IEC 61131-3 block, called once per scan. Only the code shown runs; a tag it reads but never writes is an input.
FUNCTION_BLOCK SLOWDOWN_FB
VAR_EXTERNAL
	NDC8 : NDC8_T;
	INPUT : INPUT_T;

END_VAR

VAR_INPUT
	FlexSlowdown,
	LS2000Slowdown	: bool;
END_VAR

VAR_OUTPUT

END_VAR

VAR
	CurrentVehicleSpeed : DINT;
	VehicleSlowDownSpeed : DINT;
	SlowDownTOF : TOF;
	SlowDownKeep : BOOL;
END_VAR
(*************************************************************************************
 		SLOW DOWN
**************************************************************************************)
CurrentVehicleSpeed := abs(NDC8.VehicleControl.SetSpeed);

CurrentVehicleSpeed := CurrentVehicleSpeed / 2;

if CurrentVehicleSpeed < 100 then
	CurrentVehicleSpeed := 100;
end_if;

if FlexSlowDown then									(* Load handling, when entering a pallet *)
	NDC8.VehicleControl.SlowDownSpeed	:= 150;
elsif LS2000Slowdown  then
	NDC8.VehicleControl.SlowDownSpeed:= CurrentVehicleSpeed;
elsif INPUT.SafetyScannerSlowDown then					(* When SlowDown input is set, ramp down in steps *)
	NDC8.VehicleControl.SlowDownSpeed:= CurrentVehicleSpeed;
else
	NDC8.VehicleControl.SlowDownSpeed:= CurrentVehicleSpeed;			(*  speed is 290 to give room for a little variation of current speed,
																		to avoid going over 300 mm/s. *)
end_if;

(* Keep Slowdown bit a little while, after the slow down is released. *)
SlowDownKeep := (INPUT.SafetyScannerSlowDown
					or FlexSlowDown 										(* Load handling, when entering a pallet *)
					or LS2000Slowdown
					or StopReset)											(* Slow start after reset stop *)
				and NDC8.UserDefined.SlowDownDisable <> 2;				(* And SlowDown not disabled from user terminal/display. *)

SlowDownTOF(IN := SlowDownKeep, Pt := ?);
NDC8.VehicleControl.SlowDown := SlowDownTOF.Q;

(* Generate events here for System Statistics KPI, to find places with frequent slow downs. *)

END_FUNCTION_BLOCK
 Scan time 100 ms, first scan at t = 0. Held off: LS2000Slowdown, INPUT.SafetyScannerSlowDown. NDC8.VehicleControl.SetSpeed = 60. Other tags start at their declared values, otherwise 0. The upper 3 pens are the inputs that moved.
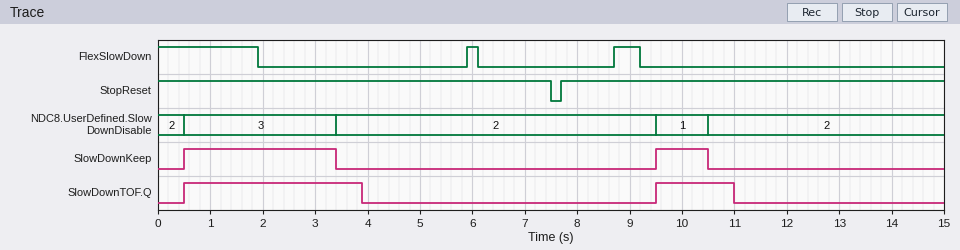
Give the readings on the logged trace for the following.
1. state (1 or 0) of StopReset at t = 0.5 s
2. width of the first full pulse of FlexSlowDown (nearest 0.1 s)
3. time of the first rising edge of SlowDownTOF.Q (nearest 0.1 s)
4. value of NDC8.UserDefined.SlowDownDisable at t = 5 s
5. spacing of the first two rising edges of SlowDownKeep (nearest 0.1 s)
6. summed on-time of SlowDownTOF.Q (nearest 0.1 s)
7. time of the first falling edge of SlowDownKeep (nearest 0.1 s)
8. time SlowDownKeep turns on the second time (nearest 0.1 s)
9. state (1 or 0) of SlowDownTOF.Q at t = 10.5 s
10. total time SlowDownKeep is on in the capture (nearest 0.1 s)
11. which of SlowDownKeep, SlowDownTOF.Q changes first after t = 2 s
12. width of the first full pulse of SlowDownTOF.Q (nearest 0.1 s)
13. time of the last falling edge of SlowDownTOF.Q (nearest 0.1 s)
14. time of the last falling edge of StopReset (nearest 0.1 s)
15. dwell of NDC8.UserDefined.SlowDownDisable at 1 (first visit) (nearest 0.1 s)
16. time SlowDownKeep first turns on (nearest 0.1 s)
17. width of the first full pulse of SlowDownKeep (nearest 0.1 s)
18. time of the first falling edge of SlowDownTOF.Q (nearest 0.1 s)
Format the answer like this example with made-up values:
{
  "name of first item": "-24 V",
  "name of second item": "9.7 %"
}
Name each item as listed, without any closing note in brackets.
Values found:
{
  "state (1 or 0) of StopReset at t = 0.5 s": "1",
  "width of the first full pulse of FlexSlowDown": "0.2 s",
  "time of the first rising edge of SlowDownTOF.Q": "0.5 s",
  "value of NDC8.UserDefined.SlowDownDisable at t = 5 s": "2",
  "spacing of the first two rising edges of SlowDownKeep": "9.0 s",
  "summed on-time of SlowDownTOF.Q": "4.9 s",
  "time of the first falling edge of SlowDownKeep": "3.4 s",
  "time SlowDownKeep turns on the second time": "9.5 s",
  "state (1 or 0) of SlowDownTOF.Q at t = 10.5 s": "1",
  "total time SlowDownKeep is on in the capture": "3.9 s",
  "which of SlowDownKeep, SlowDownTOF.Q changes first after t = 2 s": "SlowDownKeep",
  "width of the first full pulse of SlowDownTOF.Q": "3.4 s",
  "time of the last falling edge of SlowDownTOF.Q": "11.0 s",
  "time of the last falling edge of StopReset": "7.5 s",
  "dwell of NDC8.UserDefined.SlowDownDisable at 1 (first visit)": "1.0 s",
  "time SlowDownKeep first turns on": "0.5 s",
  "width of the first full pulse of SlowDownKeep": "2.9 s",
  "time of the first falling edge of SlowDownTOF.Q": "3.9 s"
}
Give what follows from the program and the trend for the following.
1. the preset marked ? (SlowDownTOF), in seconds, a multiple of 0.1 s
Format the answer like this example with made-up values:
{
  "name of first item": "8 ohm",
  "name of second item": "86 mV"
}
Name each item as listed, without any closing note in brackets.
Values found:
{
  "the preset marked ? (SlowDownTOF), in seconds, a multiple of 0.1 s": "0.5 s"
}
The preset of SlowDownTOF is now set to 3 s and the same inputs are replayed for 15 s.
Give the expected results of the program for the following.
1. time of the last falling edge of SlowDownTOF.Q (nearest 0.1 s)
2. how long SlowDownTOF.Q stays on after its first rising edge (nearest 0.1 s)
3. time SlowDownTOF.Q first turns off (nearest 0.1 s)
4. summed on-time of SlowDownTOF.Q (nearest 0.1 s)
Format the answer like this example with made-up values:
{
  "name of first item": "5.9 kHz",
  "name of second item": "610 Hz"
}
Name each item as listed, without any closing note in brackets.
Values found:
{
  "time of the last falling edge of SlowDownTOF.Q": "13.5 s",
  "how long SlowDownTOF.Q stays on after its first rising edge": "5.9 s",
  "time SlowDownTOF.Q first turns off": "6.4 s",
  "summed on-time of SlowDownTOF.Q": "9.9 s"
}
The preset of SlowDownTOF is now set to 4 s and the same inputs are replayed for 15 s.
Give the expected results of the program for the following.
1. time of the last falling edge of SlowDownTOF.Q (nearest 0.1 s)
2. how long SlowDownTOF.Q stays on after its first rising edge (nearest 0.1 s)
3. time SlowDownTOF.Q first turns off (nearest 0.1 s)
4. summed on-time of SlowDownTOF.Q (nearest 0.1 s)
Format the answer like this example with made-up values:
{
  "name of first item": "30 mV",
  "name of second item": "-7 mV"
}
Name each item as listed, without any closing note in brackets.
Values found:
{
  "time of the last falling edge of SlowDownTOF.Q": "14.5 s",
  "how long SlowDownTOF.Q stays on after its first rising edge": "6.9 s",
  "time SlowDownTOF.Q first turns off": "7.4 s",
  "summed on-time of SlowDownTOF.Q": "11.9 s"
}
